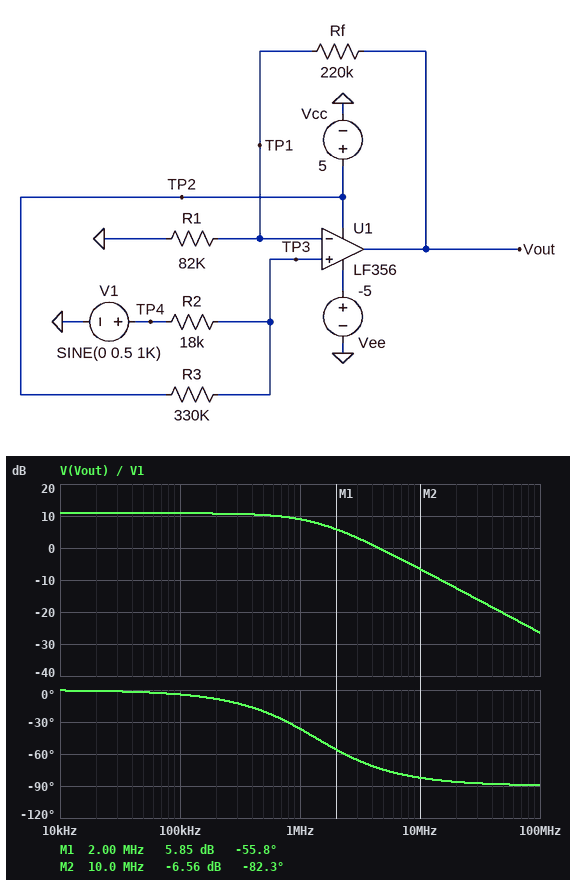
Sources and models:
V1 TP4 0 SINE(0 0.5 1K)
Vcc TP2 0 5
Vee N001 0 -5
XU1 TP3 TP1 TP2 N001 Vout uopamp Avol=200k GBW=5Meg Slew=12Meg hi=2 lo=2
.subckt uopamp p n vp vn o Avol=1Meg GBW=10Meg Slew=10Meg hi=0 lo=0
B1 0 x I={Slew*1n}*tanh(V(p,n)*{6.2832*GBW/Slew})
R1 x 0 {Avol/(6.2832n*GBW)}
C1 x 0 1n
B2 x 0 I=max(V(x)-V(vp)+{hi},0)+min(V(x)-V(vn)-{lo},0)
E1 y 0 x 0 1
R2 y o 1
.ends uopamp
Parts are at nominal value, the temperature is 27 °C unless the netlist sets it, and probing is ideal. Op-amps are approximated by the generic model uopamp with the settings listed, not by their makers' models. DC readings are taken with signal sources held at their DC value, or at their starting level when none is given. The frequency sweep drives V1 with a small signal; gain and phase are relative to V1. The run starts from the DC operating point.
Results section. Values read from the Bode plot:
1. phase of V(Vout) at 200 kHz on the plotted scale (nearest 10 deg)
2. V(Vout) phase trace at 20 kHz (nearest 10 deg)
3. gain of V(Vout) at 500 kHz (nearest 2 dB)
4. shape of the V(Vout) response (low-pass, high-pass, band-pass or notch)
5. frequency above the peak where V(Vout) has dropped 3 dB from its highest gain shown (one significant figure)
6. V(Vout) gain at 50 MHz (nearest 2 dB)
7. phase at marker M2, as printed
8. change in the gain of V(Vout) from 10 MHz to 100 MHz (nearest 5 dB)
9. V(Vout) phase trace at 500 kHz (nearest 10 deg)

-10 deg
0 deg
10 dB
low-pass
1 MHz
-20 dB
-82.3 deg
-20 dB
-20 deg
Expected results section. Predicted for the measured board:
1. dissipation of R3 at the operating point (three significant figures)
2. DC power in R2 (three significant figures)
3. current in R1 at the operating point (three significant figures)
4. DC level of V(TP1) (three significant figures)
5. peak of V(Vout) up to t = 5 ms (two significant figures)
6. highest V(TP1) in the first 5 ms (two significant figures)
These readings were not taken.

68.1 µW
3.72 µW
3.15 µA
259 mV
2.7 V
730 mV
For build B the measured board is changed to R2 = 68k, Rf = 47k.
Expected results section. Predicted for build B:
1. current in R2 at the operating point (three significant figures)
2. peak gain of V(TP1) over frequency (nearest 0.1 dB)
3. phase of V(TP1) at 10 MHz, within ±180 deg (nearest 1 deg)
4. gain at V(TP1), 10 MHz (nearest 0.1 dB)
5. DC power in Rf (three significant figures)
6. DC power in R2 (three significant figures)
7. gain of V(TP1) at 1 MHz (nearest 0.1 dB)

12.6 µA
-1.6 dB
-72 deg
-12.0 dB
5.10 µW
10.7 µW
-2.0 dB
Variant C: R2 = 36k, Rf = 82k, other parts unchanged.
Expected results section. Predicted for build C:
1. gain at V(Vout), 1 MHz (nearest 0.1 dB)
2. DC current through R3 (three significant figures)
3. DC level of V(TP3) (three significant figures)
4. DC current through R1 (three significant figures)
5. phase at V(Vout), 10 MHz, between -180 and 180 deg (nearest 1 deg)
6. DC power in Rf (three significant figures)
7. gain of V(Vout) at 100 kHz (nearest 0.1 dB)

4.5 dB
13.7 µA
492 mV
6.00 µA
-76 deg
2.95 µW
5.1 dB
